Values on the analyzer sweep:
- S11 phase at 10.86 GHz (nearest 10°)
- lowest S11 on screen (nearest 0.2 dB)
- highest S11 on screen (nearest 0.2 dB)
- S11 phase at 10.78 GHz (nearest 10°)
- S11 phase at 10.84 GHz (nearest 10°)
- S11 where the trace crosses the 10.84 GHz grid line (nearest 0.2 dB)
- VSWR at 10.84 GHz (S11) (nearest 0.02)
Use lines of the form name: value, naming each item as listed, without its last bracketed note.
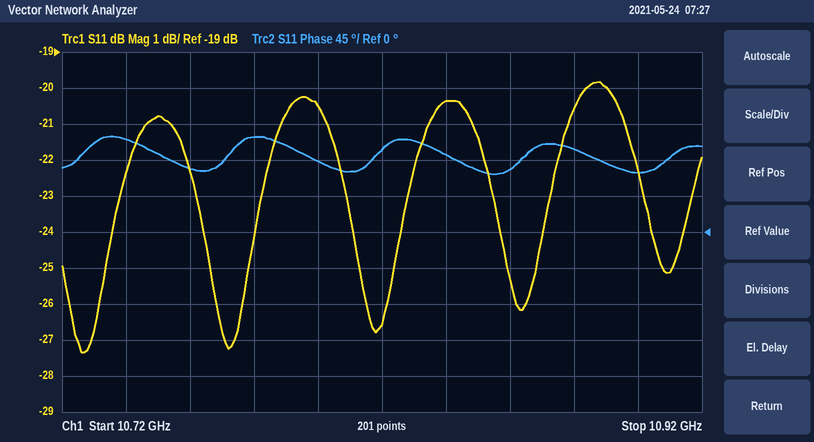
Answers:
S11 phase at 10.86 GHz: 80°
lowest S11 on screen: -27.4 dB
highest S11 on screen: -19.8 dB
S11 phase at 10.78 GHz: 120°
S11 phase at 10.84 GHz: 100°
S11 where the trace crosses the 10.84 GHz grid line: -20.4 dB
VSWR at 10.84 GHz (S11): 1.22
